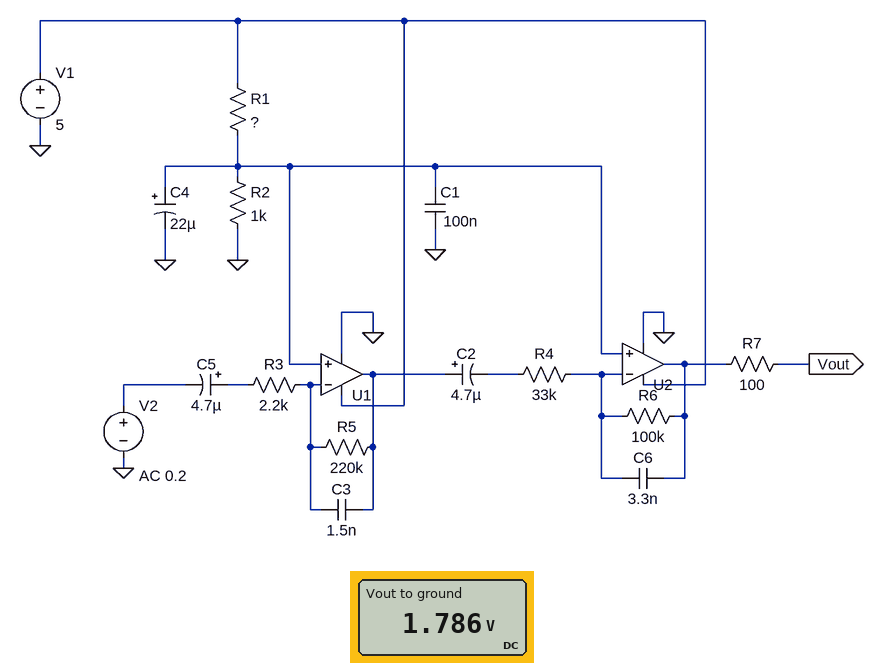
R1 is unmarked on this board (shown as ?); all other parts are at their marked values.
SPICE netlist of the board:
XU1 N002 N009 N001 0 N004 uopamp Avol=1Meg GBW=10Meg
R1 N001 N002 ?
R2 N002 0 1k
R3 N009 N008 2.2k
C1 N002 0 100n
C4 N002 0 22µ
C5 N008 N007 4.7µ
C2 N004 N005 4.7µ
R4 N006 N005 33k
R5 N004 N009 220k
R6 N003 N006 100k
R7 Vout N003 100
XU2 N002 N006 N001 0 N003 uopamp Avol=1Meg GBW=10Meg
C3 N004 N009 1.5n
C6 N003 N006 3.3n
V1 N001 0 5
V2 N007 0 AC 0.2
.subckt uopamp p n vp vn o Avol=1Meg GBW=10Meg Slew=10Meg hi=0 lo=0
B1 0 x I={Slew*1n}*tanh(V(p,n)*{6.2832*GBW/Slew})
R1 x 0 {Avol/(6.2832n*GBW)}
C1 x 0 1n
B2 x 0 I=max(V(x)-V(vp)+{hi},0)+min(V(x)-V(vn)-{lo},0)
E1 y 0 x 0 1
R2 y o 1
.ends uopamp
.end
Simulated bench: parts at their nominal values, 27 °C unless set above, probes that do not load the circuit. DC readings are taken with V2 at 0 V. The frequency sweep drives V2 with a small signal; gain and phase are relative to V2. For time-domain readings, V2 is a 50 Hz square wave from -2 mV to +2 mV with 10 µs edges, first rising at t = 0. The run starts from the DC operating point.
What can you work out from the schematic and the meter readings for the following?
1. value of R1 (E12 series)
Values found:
1.8 kΩ
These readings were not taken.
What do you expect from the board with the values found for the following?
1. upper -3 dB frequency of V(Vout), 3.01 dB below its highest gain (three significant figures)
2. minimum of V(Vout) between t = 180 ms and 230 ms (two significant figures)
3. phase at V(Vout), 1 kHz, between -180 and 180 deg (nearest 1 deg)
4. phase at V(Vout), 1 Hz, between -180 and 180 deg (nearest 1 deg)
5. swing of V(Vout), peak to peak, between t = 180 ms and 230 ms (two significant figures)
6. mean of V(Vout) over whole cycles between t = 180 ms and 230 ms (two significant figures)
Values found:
332 Hz
1.0 V
-128 deg
132 deg
1.5 V
1.8 V
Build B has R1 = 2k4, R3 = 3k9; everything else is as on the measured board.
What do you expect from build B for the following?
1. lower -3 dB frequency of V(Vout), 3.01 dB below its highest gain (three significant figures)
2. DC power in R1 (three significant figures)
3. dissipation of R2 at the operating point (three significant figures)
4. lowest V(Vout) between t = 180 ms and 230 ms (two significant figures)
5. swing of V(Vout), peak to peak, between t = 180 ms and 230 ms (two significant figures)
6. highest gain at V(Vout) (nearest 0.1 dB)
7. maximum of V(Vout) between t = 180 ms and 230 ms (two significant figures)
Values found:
8.39 Hz
5.19 mW
2.16 mW
1.1 V
800 mV
44.4 dB
1.9 V
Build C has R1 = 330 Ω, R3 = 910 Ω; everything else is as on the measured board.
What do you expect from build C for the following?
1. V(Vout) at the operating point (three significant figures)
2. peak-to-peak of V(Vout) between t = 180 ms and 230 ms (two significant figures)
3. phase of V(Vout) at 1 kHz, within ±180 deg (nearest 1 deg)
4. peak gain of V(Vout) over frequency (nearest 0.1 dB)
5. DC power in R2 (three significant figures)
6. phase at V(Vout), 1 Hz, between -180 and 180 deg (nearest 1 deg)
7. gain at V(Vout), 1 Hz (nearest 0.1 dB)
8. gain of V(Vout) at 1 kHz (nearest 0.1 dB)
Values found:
3.76 V
3.3 V
-127 deg
56.4 dB
14.1 mW
134 deg
22.8 dB
42.7 dB
